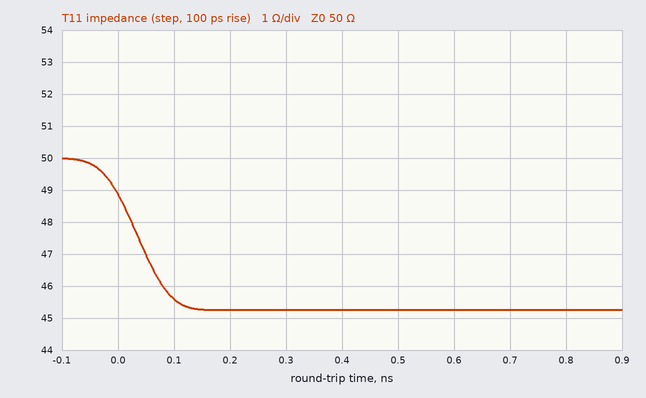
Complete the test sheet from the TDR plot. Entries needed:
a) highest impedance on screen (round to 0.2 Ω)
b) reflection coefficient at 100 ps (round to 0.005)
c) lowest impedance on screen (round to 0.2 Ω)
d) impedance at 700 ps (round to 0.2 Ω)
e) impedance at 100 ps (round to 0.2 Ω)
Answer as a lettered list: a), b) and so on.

a) 50.0 Ω
b) -0.045
c) 45.2 Ω
d) 45.2 Ω
e) 45.6 Ω
